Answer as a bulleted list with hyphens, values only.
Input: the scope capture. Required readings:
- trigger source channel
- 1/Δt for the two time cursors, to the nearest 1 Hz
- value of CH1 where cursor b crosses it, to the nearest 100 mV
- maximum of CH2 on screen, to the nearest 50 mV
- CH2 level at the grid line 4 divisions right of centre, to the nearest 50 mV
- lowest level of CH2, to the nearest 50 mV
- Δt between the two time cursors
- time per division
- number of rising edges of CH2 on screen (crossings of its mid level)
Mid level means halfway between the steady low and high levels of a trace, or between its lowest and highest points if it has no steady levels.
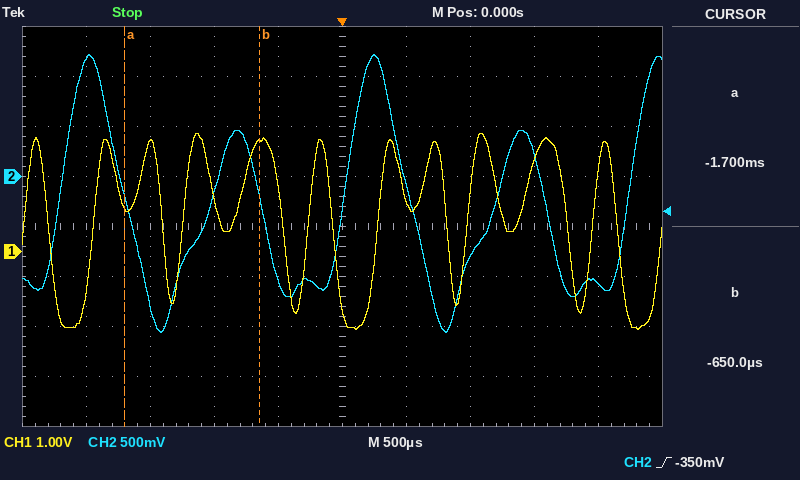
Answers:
- CH2
- 952 Hz
- 2.2 V
- 1.20 V
- -1.05 V
- -1.55 V
- 1.05 ms
- 500 µs
- 5
